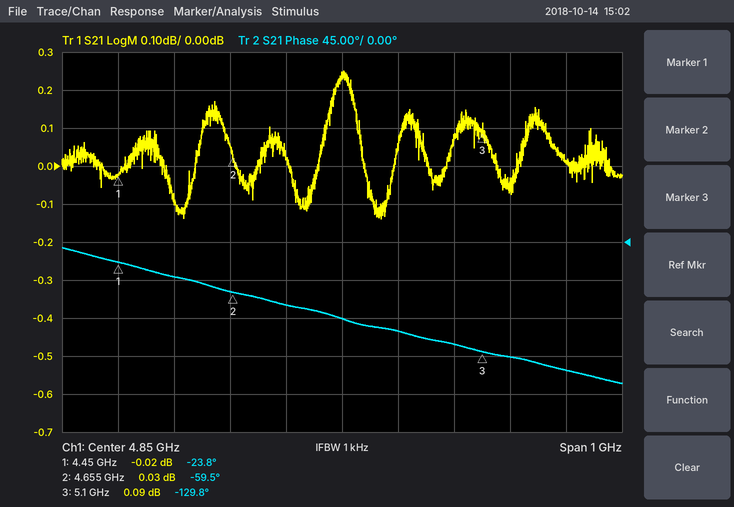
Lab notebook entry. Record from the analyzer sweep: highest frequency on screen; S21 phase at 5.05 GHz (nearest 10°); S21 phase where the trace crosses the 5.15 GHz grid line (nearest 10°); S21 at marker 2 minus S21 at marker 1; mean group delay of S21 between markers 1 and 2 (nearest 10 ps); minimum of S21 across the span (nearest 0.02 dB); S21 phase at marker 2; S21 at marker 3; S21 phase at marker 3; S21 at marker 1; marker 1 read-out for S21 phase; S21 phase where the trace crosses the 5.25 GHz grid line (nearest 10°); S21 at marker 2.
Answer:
5.35 GHz
-120°
-140°
0.05 dB
480 ps
-0.14 dB
-59.5°
0.09 dB
-129.8°
-0.02 dB
-23.8°
-150°
0.03 dB
